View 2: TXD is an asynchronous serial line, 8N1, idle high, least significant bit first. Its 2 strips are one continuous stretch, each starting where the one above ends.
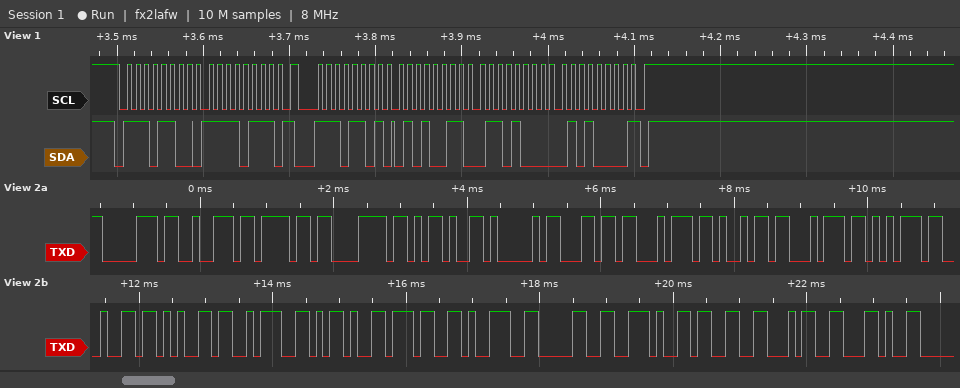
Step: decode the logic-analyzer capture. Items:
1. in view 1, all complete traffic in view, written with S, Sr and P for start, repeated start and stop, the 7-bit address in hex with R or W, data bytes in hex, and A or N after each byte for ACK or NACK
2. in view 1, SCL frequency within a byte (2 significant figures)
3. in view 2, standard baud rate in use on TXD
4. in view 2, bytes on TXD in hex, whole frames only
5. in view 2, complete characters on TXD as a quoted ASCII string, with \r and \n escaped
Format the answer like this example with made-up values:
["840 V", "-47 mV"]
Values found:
["S 76W A F7 A Sr 76R A 53 A 68 A 50 N P", "100 kHz", "9600 baud", "0x70 0x72 0x6F 0x78 0x2D 0x41 0x6C 0x74 0x69 0x74 0x75 0x64 0x65 0x3A 0x2D 0x37 0x39 0x30 0x2E 0x33 0x34 0x2C", "\"prox-Altitude:-790.34,\""]
